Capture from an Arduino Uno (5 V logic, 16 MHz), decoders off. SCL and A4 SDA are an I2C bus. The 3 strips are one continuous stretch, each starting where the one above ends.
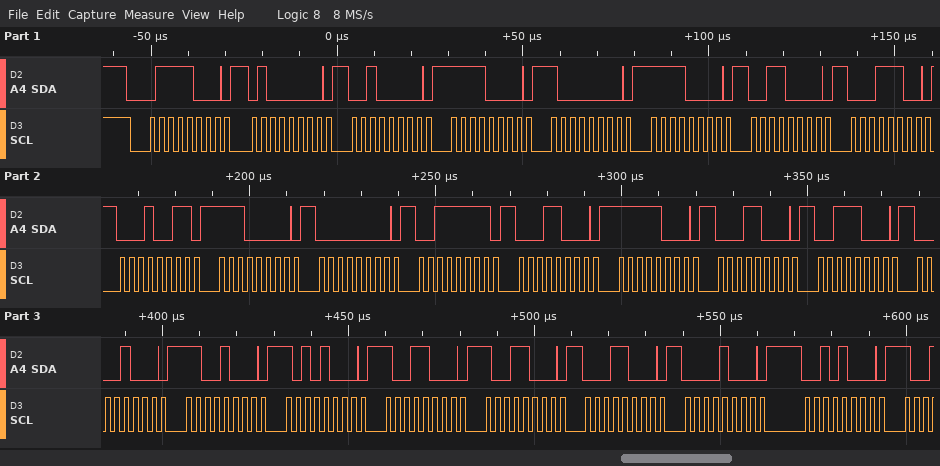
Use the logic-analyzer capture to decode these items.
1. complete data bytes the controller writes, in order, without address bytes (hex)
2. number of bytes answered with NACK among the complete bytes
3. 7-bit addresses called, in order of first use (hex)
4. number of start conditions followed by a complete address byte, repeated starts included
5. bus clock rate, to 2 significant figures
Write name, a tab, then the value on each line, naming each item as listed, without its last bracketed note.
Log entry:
complete data bytes the controller writes, in order, without address bytes	40 20 F0 80 F0 30 1C 13 E0 00 3F 18 F8 18 38 08 C8 A8 98 98 18 08 28
number of bytes answered with NACK among the complete bytes	0
7-bit addresses called, in order of first use	0x3C
number of start conditions followed by a complete address byte, repeated starts included	1
bus clock rate, to 2 significant figures	400 kHz
